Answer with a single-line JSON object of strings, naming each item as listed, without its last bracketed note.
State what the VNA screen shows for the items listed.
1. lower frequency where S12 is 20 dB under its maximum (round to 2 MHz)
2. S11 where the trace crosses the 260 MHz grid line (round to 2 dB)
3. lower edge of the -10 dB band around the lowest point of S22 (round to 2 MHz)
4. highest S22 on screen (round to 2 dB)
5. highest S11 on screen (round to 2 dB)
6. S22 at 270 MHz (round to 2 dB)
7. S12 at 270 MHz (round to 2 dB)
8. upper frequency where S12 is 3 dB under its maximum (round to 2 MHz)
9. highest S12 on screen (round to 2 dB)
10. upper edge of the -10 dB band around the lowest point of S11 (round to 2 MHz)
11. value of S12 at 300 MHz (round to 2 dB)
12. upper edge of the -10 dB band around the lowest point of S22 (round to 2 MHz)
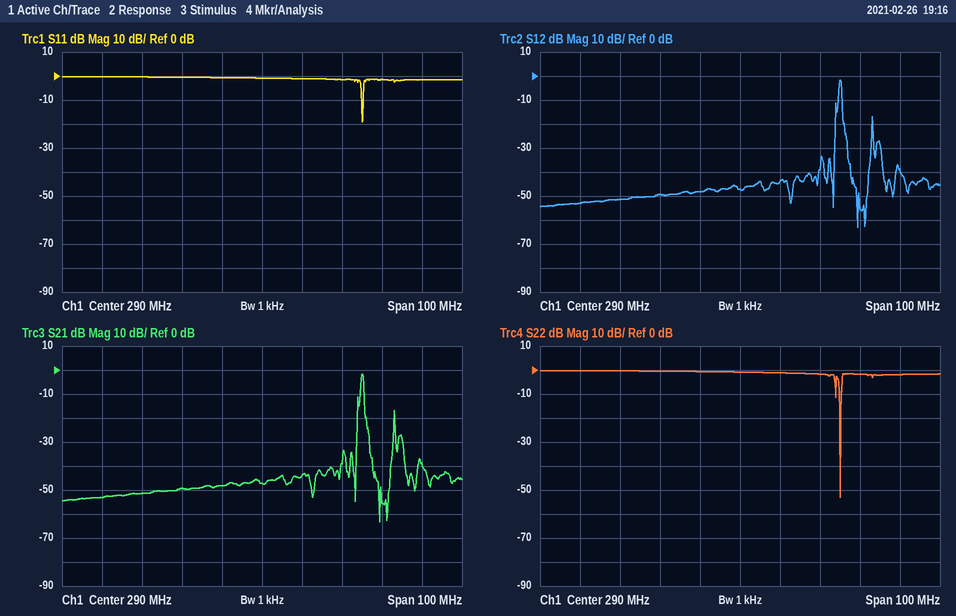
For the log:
{"lower frequency where S12 is 20 dB under its maximum": "314 MHz", "S11 where the trace crosses the 260 MHz grid line": "0 dB", "lower edge of the -10 dB band around the lowest point of S22": "314 MHz", "highest S22 on screen": "0 dB", "highest S11 on screen": "0 dB", "S22 at 270 MHz": "0 dB", "S12 at 270 MHz": "-50 dB", "upper frequency where S12 is 3 dB under its maximum": "316 MHz", "highest S12 on screen": "-2 dB", "upper edge of the -10 dB band around the lowest point of S11": "316 MHz", "value of S12 at 300 MHz": "-44 dB", "upper edge of the -10 dB band around the lowest point of S22": "316 MHz"}
